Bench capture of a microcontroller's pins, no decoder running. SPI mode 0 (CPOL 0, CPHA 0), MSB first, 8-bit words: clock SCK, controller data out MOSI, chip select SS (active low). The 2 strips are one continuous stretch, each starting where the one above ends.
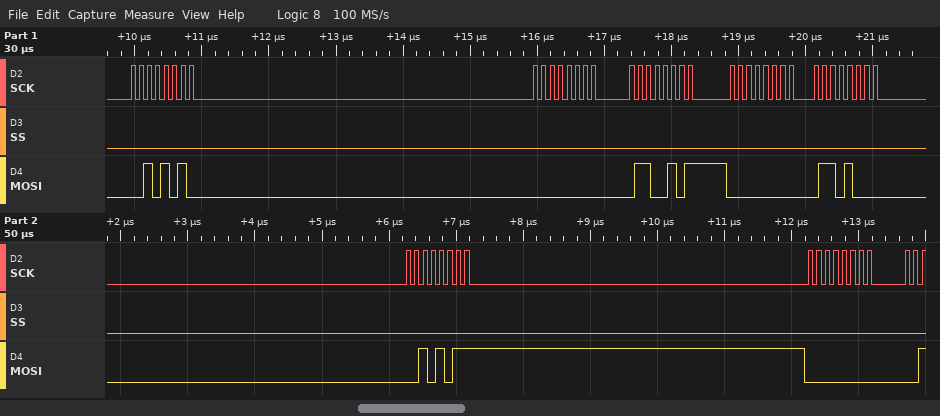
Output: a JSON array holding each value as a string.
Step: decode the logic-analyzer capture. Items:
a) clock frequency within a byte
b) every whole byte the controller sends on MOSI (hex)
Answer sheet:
["8 MHz", "2A 00 65 00 68 2B 00"]
